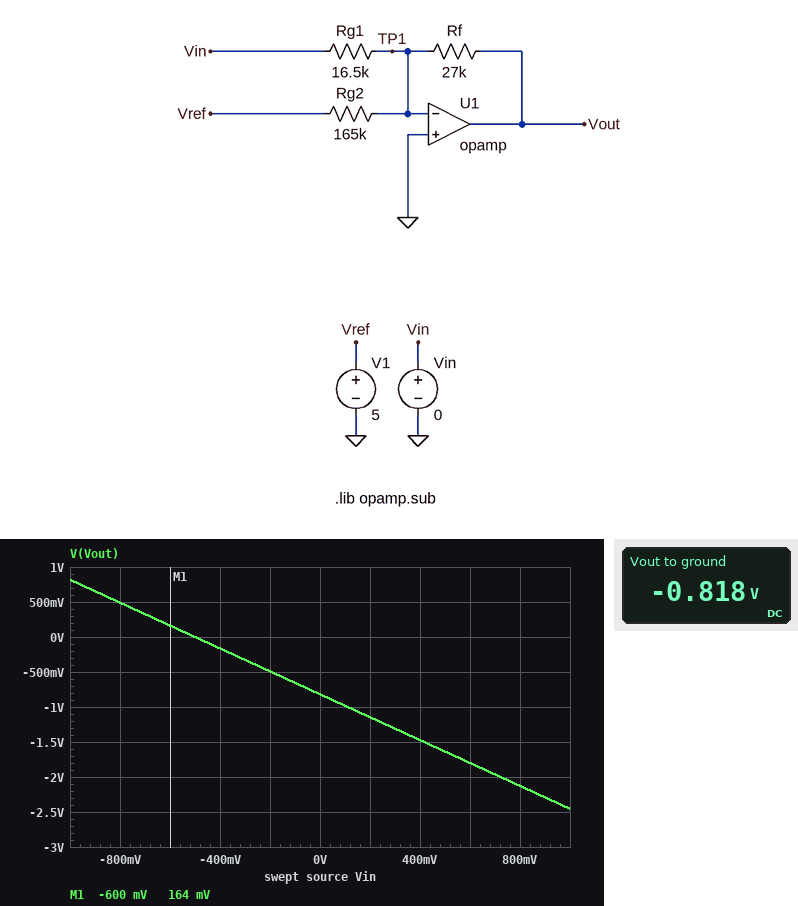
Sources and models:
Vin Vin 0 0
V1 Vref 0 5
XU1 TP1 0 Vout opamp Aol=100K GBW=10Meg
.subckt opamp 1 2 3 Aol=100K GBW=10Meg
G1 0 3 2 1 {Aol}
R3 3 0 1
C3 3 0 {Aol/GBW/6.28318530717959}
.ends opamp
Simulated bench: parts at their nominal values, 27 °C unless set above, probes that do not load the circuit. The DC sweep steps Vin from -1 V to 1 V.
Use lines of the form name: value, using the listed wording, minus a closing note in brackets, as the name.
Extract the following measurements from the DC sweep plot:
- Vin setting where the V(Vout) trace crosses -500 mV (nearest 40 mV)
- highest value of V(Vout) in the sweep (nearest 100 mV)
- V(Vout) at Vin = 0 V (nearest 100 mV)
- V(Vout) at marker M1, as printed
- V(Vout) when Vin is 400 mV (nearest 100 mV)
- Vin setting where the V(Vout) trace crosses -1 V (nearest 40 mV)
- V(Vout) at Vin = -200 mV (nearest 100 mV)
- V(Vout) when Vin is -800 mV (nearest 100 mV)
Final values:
Vin setting where the V(Vout) trace crosses -500 mV: -200 mV
highest value of V(Vout) in the sweep: 800 mV
V(Vout) at Vin = 0 V: -800 mV
V(Vout) at marker M1, as printed: 164 mV
V(Vout) when Vin is 400 mV: -1.5 V
Vin setting where the V(Vout) trace crosses -1 V: 120 mV
V(Vout) at Vin = -200 mV: -500 mV
V(Vout) when Vin is -800 mV: 500 mV
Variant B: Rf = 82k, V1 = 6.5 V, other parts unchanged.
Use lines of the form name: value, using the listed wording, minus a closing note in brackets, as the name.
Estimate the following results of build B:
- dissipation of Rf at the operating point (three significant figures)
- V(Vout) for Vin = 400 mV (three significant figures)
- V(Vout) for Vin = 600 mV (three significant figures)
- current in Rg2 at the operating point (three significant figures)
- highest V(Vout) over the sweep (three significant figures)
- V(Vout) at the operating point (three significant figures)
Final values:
dissipation of Rf at the operating point: 127 µW
V(Vout) for Vin = 400 mV: -5.22 V
V(Vout) for Vin = 600 mV: -6.21 V
current in Rg2 at the operating point: 39.4 µA
highest V(Vout) over the sweep: 1.74 V
V(Vout) at the operating point: -3.23 V
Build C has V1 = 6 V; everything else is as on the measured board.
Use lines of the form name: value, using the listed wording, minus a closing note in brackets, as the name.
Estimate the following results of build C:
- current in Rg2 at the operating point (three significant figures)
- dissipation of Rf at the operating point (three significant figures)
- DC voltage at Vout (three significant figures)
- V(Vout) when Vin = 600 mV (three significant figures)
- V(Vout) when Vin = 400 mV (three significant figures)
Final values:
current in Rg2 at the operating point: 36.4 µA
dissipation of Rf at the operating point: 35.7 µW
DC voltage at Vout: -982 mV
V(Vout) when Vin = 600 mV: -1.96 V
V(Vout) when Vin = 400 mV: -1.64 V
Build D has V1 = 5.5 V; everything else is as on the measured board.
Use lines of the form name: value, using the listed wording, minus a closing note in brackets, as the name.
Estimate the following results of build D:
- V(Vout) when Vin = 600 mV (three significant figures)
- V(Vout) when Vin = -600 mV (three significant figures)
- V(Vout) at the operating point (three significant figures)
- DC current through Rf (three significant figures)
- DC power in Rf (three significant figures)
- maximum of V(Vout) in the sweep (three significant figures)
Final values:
V(Vout) when Vin = 600 mV: -1.88 V
V(Vout) when Vin = -600 mV: 81.8 mV
V(Vout) at the operating point: -900 mV
DC current through Rf: 33.3 µA
DC power in Rf: 30.0 µW
maximum of V(Vout) in the sweep: 736 mV
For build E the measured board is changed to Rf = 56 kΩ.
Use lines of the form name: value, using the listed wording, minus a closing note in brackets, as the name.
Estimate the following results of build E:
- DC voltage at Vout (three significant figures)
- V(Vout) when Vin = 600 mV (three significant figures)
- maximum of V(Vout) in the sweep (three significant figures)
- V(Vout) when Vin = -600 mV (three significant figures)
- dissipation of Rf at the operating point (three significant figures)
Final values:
DC voltage at Vout: -1.70 V
V(Vout) when Vin = 600 mV: -3.73 V
maximum of V(Vout) in the sweep: 1.70 V
V(Vout) when Vin = -600 mV: 339 mV
dissipation of Rf at the operating point: 51.4 µW
